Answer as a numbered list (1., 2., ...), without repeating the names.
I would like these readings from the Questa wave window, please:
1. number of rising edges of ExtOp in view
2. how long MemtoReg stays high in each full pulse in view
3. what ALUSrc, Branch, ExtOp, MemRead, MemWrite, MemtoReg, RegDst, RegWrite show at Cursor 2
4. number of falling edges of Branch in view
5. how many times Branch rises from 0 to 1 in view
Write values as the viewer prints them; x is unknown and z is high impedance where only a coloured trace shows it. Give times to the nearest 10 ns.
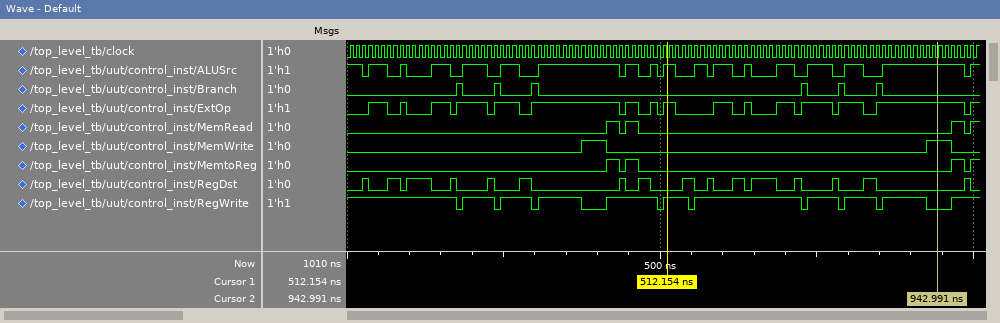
1. 16
2. 20 ns, 20 ns, 20 ns
3. ALUSrc=1, Branch=0, ExtOp=1, MemRead=0, MemWrite=1, MemtoReg=0, RegDst=0, RegWrite=0
4. 6
5. 6
